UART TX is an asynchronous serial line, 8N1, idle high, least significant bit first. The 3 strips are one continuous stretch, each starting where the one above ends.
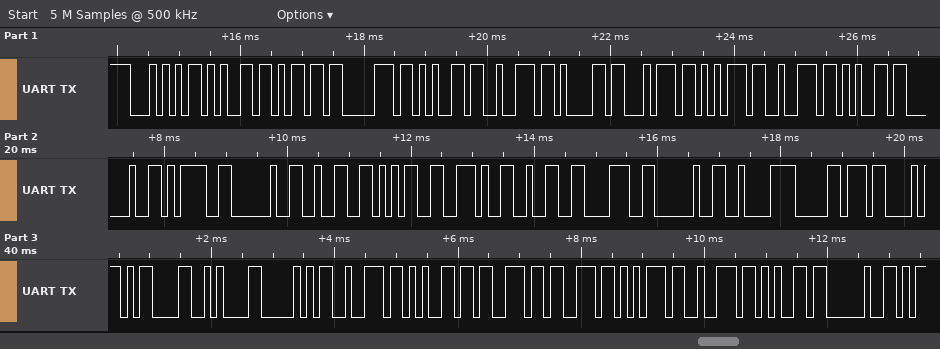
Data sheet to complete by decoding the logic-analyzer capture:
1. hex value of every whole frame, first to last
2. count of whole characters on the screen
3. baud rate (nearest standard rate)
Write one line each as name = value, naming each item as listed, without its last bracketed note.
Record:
hex value of every whole frame, first to last = 0x54 0x65 0x6D 0x70 0x65 0x72 0x61 0x74 0x75 0x72 0x65 0x20 0x3D 0x20 0x32 0x35 0x2E 0x32 0x38 0x20 0xC2 0xB0 0x43 0x0D 0x0A 0x50 0x72 0x65 0x73 0x73 0x75 0x72 0x65 0x20
count of whole characters on the screen = 34
baud rate = 9600 baud
